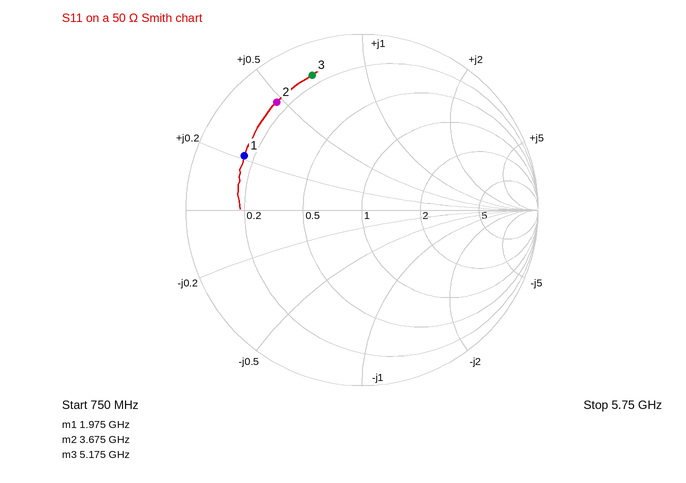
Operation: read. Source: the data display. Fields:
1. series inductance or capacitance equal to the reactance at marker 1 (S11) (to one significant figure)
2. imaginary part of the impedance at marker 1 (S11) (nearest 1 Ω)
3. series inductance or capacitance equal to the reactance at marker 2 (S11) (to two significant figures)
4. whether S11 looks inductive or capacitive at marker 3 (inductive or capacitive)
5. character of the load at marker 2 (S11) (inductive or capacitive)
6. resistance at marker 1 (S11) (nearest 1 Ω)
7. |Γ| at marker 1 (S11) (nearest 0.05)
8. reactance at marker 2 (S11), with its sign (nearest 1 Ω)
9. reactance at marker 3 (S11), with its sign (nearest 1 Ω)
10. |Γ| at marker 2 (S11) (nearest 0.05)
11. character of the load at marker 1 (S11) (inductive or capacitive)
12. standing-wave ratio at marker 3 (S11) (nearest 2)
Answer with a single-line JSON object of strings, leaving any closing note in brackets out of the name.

{"series inductance or capacitance equal to the reactance at marker 1 (S11)": "900 pH", "imaginary part of the impedance at marker 1 (S11)": "+11 Ω", "series inductance or capacitance equal to the reactance at marker 2 (S11)": "1.0 nH", "whether S11 looks inductive or capacitive at marker 3": "inductive", "character of the load at marker 2 (S11)": "inductive", "resistance at marker 1 (S11)": "8 Ω", "|Γ| at marker 1 (S11)": "0.75", "reactance at marker 2 (S11), with its sign": "+24 Ω", "reactance at marker 3 (S11), with its sign": "+34 Ω", "|Γ| at marker 2 (S11)": "0.80", "character of the load at marker 1 (S11)": "inductive", "standing-wave ratio at marker 3 (S11)": "10"}
